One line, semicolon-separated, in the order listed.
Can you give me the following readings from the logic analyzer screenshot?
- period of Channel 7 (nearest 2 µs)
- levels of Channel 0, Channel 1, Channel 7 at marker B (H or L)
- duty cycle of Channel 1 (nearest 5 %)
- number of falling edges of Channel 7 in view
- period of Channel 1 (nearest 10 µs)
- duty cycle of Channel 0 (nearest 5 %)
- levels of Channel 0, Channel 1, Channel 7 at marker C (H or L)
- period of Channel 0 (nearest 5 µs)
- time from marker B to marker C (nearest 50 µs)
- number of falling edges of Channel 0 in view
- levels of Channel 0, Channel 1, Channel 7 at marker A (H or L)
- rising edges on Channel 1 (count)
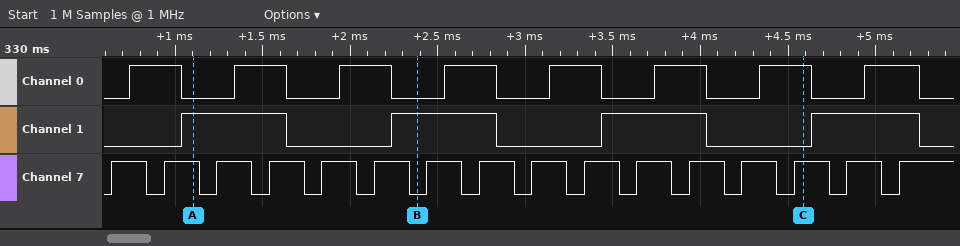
300 µs; Channel 0=L, Channel 1=H, Channel 7=L; 50 %; 15; 1200 µs; 50 %; Channel 0=H, Channel 1=L, Channel 7=H; 600 µs; 2200 µs; 8; Channel 0=L, Channel 1=H, Channel 7=H; 4
